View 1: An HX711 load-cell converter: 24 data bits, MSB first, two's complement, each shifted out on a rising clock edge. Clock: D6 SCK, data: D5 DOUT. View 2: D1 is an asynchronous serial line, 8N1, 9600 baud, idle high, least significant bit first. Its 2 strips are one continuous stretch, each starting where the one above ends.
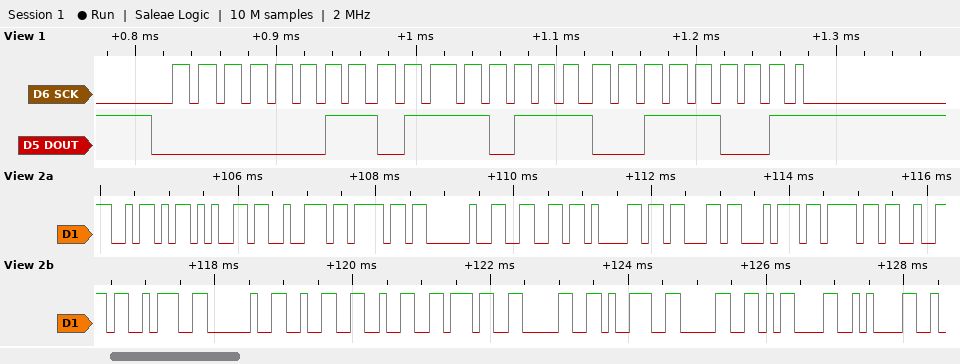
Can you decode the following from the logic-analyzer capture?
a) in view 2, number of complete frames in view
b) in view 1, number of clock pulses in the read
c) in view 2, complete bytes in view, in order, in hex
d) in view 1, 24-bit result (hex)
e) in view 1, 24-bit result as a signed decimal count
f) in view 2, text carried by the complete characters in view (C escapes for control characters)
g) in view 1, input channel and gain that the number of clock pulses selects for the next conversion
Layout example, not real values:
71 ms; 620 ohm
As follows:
21; 25; 5A 65 72 6F 20 66 61 63 74 6F 72 3A 20 32 32 37 30 39 30 0D 0A; 0x037739; 227129; "Zero factor: 227090\r\n"; channel A, gain 128
